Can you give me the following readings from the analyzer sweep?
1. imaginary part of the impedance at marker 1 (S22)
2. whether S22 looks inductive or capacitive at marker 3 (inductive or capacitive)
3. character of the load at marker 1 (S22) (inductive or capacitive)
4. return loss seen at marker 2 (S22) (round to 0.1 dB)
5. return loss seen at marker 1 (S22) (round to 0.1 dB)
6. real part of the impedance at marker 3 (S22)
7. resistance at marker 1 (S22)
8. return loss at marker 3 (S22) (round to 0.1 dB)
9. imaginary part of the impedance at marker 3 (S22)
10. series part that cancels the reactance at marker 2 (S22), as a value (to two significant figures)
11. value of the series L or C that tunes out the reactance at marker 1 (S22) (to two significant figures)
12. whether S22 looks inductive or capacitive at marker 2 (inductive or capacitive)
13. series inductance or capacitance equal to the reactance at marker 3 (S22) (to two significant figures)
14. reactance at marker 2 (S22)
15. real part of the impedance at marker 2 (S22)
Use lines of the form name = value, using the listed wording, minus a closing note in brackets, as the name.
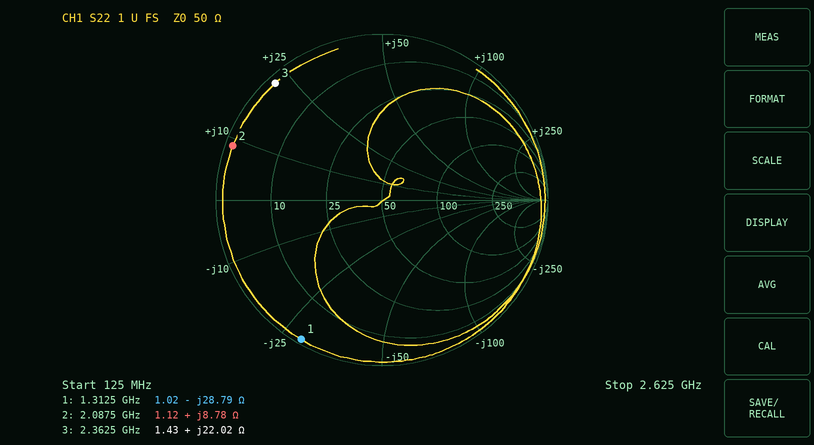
imaginary part of the impedance at marker 1 = -28.79 Ω
whether S22 looks inductive or capacitive at marker 3 = inductive
character of the load at marker 1 (S22) = capacitive
return loss seen at marker 2 (S22) = 0.4 dB
return loss seen at marker 1 (S22) = 0.3 dB
real part of the impedance at marker 3 = 1.43 Ω
resistance at marker 1 = 1.02 Ω
return loss at marker 3 (S22) = 0.4 dB
imaginary part of the impedance at marker 3 = +22.02 Ω
series part that cancels the reactance at marker 2 (S22), as a value = 8.7 pF
value of the series L or C that tunes out the reactance at marker 1 (S22) = 3.5 nH
whether S22 looks inductive or capacitive at marker 2 = inductive
series inductance or capacitance equal to the reactance at marker 3 (S22) = 1.5 nH
reactance at marker 2 = +8.78 Ω
real part of the impedance at marker 2 = 1.12 Ω
